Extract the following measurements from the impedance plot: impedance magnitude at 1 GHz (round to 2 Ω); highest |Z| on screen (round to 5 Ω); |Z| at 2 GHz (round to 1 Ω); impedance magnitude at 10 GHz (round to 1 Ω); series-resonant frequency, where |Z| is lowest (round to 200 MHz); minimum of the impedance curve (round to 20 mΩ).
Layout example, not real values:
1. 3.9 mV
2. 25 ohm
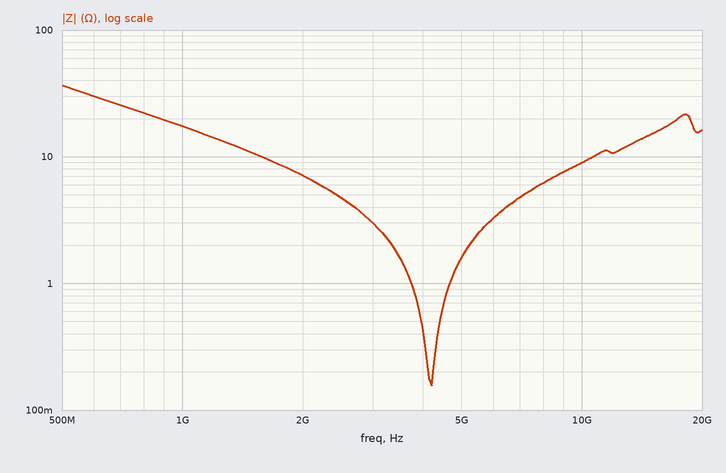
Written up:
1. 18 Ω
2. 35 Ω
3. 7 Ω
4. 9 Ω
5. 4.2 GHz
6. 160 mΩ
